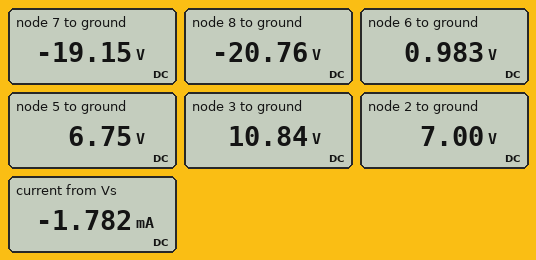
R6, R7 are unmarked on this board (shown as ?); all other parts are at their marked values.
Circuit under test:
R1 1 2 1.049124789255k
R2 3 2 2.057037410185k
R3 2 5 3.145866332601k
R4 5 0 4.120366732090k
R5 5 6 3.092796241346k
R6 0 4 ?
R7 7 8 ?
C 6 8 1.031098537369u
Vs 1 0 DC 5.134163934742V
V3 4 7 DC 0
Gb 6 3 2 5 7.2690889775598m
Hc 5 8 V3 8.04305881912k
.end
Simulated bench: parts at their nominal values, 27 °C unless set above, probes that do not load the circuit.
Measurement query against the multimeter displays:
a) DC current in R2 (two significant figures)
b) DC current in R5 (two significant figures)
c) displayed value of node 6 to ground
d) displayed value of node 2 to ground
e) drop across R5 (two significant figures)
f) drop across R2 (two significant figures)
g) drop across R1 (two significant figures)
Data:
1.9 mA
1.9 mA
0.983 V
7.00 V
5.8 V
3.8 V
1.9 V
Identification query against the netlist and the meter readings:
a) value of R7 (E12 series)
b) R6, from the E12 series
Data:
470 Ω
5.6 kΩ
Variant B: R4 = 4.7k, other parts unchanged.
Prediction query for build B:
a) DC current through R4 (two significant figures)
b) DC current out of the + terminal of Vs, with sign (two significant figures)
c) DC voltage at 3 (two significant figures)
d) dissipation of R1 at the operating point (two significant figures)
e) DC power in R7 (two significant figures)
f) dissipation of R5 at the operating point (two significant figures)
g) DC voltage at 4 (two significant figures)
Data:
1.5 mA
-2.1 mA
12 V
4.4 mW
5.9 mW
14 mW
-20 V
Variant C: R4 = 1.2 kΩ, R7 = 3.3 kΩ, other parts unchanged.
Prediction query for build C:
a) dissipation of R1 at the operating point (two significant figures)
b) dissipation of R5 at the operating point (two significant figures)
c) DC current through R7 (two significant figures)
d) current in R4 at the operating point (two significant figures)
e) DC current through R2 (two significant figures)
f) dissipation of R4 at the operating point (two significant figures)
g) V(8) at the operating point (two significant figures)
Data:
14 mW
45 mW
2.1 mA
1.5 mA
3.8 mA
2.8 mW
19 V
